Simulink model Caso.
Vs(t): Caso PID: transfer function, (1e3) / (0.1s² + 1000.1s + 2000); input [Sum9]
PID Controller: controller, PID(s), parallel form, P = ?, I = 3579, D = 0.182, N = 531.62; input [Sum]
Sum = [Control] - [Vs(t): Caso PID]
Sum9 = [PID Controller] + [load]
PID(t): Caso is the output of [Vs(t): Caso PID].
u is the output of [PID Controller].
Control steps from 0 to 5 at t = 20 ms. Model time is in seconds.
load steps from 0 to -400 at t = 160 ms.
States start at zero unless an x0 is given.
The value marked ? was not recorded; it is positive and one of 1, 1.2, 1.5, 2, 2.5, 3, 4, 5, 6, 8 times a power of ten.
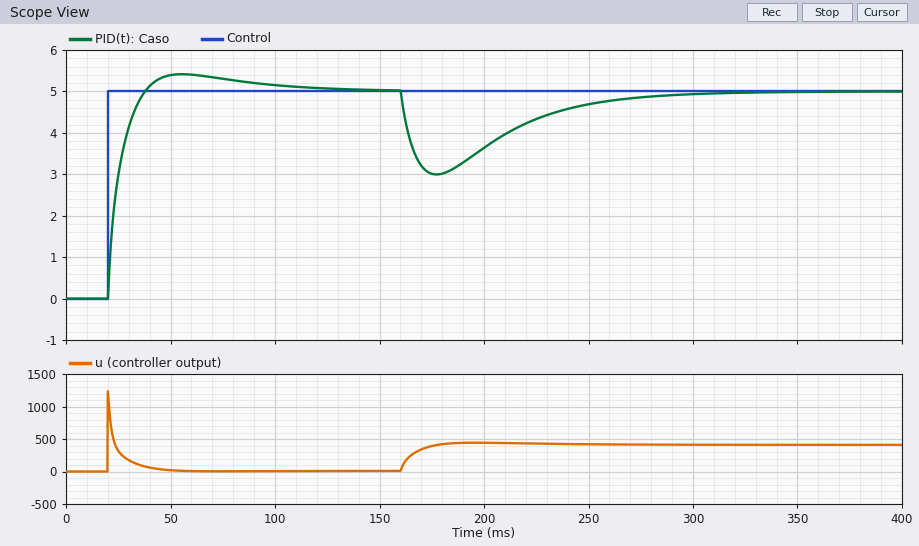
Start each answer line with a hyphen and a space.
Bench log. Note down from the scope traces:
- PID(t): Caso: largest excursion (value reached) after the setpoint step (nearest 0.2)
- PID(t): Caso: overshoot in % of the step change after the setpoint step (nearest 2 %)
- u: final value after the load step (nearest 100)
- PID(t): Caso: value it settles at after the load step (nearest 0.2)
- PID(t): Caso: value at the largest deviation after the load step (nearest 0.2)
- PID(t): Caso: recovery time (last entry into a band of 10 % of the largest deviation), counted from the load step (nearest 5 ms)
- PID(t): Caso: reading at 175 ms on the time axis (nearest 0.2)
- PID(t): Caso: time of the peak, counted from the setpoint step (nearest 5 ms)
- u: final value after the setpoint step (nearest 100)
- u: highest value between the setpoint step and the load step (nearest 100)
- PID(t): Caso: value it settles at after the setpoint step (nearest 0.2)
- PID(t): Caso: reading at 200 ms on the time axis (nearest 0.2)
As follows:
- 5.4
- 8 %
- 400
- 5.0
- 3.0
- 105 ms
- 3.0
- 35 ms
- 0
- 1200
- 5.0
- 3.6
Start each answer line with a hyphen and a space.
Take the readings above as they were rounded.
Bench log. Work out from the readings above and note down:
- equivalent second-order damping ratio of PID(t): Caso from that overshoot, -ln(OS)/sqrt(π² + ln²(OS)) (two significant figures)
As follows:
- 0.63
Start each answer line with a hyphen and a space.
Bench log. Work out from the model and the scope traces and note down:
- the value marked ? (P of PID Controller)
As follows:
- 150
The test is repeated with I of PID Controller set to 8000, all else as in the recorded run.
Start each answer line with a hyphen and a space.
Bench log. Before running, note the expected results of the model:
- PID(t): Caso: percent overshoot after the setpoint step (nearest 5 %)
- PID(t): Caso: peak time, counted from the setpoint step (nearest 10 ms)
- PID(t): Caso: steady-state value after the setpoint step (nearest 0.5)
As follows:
- 15 %
- 30 ms
- 5.0
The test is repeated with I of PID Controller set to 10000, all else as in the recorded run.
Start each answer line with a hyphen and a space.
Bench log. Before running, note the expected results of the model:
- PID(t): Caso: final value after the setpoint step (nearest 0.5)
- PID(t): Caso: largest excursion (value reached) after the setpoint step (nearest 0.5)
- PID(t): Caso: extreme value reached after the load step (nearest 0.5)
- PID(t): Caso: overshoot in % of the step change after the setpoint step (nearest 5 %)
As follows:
- 5.0
- 6.0
- 3.5
- 15 %
